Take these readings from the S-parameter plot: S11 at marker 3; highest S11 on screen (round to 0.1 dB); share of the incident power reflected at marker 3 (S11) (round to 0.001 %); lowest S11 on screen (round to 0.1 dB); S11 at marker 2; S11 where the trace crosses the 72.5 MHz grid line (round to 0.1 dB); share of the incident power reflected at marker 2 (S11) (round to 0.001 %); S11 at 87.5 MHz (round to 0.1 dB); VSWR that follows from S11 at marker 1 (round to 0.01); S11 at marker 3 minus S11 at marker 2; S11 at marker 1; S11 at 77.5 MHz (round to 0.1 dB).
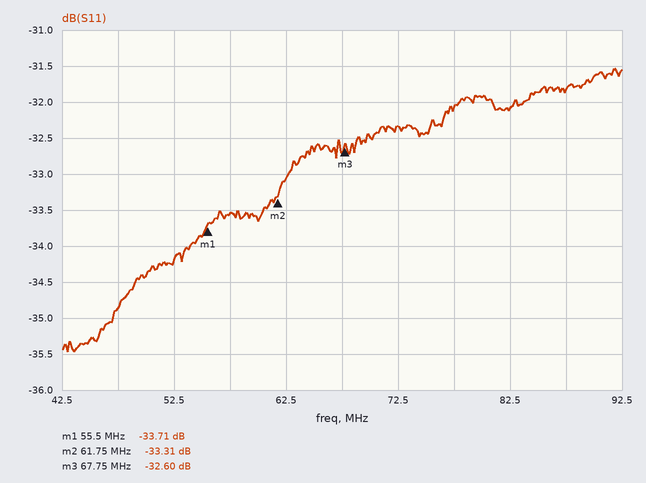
-32.60 dB
-31.5 dB
0.055 %
-35.5 dB
-33.31 dB
-32.3 dB
0.047 %
-31.8 dB
1.04
0.71 dB
-33.71 dB
-32.1 dB
